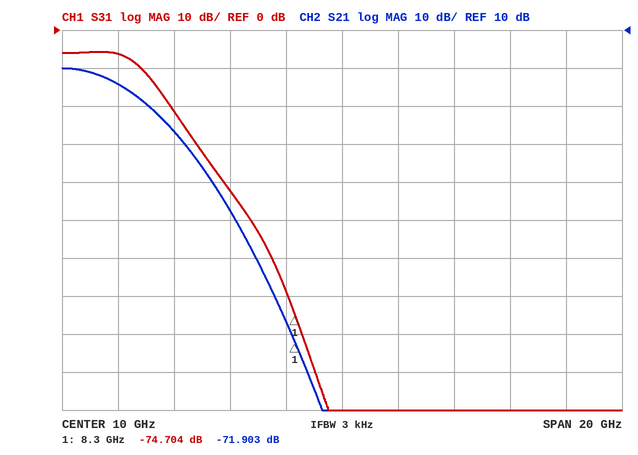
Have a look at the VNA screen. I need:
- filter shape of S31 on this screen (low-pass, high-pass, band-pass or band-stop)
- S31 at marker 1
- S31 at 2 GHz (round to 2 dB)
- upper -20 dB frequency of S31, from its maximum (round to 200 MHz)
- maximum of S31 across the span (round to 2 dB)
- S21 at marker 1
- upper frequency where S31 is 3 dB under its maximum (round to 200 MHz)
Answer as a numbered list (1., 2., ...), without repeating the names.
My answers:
1. low-pass
2. -74.704 dB
3. -6 dB
4. 4.4 GHz
5. -6 dB
6. -71.903 dB
7. 2.6 GHz
